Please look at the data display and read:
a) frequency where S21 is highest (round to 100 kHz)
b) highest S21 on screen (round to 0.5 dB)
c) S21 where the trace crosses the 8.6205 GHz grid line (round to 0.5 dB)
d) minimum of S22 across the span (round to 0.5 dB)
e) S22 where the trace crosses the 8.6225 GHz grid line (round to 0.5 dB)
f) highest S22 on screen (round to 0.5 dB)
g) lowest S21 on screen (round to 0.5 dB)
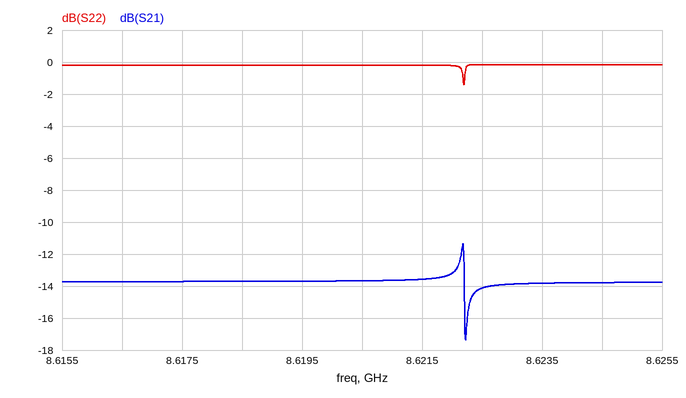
8.6222 GHz
-11.5 dB
-13.5 dB
-1.5 dB
0.0 dB
0.0 dB
-17.5 dB
